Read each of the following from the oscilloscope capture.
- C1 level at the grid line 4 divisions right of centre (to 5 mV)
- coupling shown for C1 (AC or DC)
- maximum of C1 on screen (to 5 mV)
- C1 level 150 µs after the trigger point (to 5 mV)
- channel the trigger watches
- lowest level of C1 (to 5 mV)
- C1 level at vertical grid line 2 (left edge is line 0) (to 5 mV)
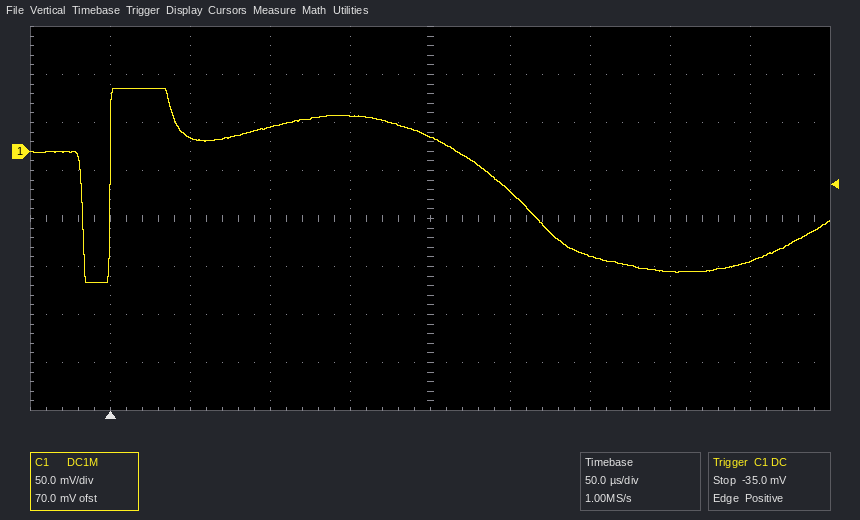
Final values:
-115 mV
DC
65 mV
35 mV
C1
-135 mV
15 mV
